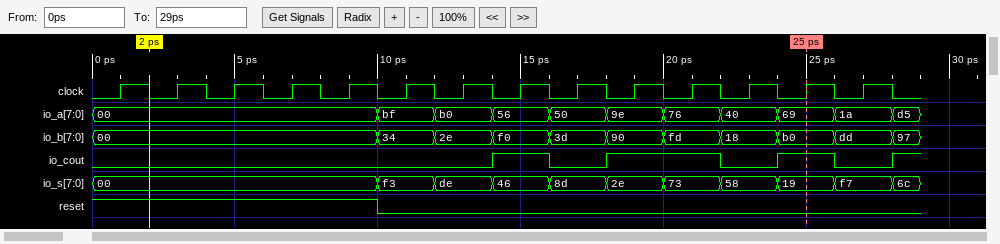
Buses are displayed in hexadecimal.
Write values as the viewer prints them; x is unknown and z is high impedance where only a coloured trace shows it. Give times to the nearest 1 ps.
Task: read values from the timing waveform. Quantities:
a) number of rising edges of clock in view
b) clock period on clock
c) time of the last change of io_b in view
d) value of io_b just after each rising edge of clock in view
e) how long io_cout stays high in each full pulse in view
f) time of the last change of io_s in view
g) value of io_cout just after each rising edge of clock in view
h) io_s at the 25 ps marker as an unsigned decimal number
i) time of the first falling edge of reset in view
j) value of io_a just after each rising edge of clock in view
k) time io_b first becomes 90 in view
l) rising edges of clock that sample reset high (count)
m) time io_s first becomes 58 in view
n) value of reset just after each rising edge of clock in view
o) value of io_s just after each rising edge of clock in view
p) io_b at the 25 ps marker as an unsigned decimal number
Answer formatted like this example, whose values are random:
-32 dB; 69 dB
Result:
14; 2 ps; 28 ps; 00, 00, 00, 00, 00, 34, 2e, f0, 3d, 90, fd, 18, b0, dd; 2 ps, 4 ps, 2 ps; 28 ps; 0 0 0 0 0 0 0 1 0 1 1 0 1 0; 25; 10 ps; 00, 00, 00, 00, 00, bf, b0, 56, 50, 9e, 76, 40, 69, 1a; 18 ps; 5; 22 ps; 1 1 1 1 1 0 0 0 0 0 0 0 0 0; 00, 00, 00, 00, 00, f3, de, 46, 8d, 2e, 73, 58, 19, f7; 176
